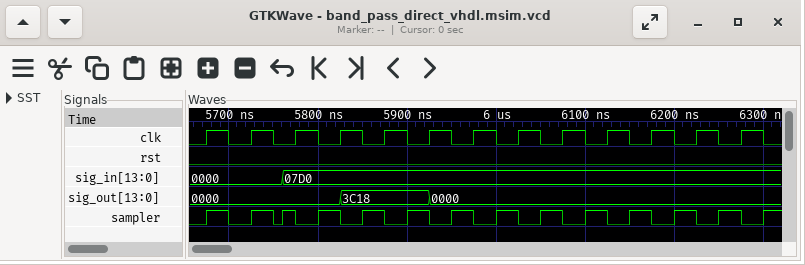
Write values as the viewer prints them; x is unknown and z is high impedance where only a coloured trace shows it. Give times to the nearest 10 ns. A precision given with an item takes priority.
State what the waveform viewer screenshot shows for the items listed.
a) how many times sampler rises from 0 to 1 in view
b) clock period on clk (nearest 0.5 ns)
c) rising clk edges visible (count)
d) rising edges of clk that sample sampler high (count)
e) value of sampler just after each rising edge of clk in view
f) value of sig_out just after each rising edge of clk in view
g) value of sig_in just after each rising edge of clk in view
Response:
14
50 ns
13
11
1 1 0 0 0 0 0 0 0 0 0 0 0
0000, 0000, 0000, 3C18, 3C18, 0000, 0000, 0000, 0000, 0000, 0000, 0000, 0000
0000, 0000, 07D0, 07D0, 07D0, 07D0, 07D0, 07D0, 07D0, 07D0, 07D0, 07D0, 07D0
